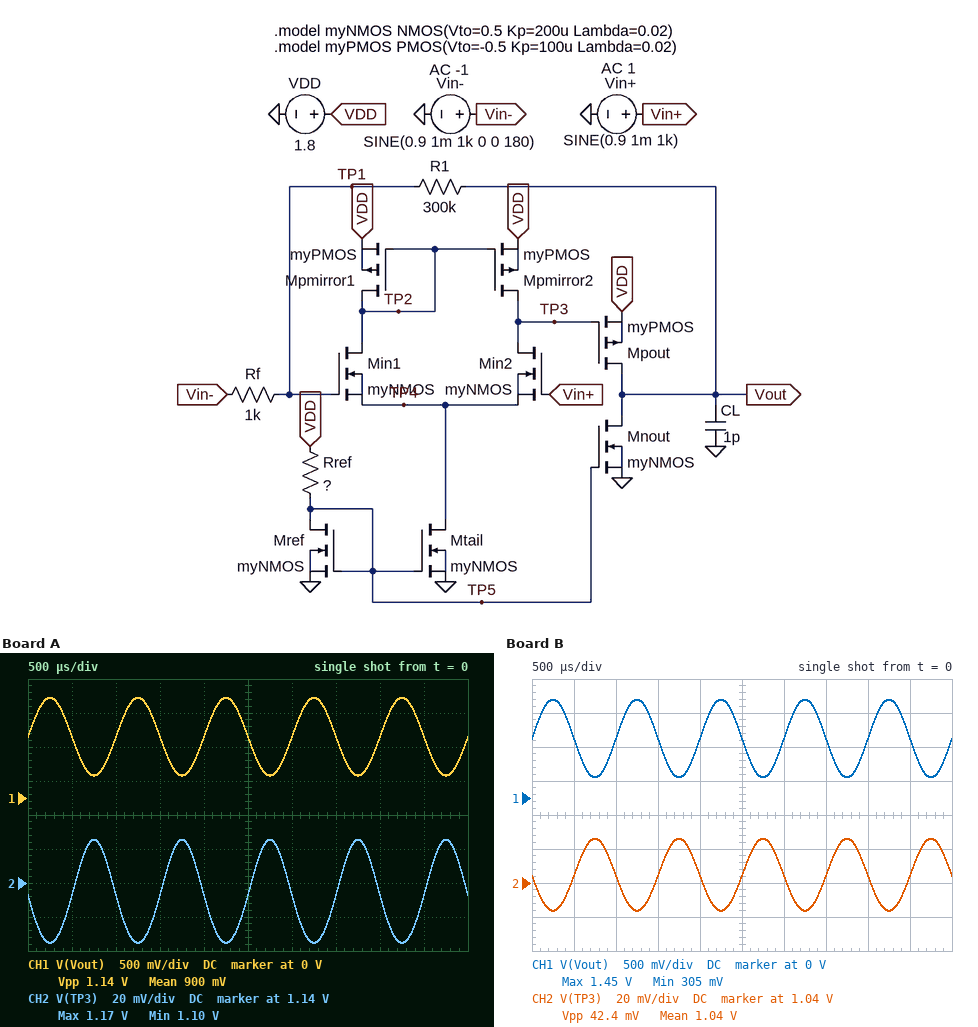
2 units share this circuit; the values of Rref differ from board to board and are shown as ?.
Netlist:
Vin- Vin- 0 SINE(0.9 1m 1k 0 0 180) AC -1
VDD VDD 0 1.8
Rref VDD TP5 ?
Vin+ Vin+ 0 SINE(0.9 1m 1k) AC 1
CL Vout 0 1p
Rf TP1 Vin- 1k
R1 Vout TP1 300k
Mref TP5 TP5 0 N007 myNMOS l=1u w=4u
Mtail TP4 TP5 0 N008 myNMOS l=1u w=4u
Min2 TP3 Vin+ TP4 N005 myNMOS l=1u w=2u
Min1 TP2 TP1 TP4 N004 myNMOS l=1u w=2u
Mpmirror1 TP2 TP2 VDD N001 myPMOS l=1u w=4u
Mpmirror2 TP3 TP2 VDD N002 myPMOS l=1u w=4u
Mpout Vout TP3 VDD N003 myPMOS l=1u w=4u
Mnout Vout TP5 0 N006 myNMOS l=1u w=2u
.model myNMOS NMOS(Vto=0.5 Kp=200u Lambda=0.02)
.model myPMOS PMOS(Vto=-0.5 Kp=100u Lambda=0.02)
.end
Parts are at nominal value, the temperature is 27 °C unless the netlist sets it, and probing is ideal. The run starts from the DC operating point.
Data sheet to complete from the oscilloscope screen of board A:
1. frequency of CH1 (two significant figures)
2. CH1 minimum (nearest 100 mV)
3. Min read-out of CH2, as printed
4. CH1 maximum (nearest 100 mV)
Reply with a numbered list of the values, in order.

1. 1.0 kHz
2. 300 mV
3. 1.10 V
4. 1.5 V
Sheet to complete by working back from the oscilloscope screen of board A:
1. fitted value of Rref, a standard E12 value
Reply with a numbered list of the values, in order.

1. 100 kΩ
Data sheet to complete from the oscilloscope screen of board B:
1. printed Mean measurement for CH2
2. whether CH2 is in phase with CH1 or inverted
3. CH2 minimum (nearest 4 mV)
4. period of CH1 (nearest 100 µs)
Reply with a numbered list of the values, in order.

1. 1.04 V
2. inverted
3. 1.024 V
4. 1.0 ms
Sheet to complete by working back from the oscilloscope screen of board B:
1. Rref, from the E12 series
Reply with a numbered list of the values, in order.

1. 39 kΩ
